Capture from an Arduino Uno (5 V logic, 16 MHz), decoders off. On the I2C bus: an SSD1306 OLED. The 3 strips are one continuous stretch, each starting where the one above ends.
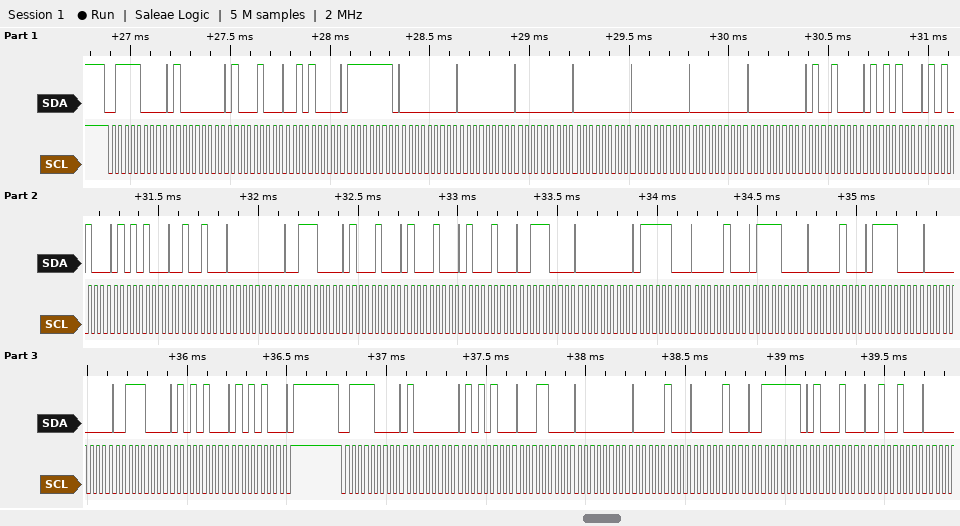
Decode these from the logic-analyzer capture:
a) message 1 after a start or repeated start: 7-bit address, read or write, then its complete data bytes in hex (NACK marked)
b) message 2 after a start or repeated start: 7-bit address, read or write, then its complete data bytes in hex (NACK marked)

0x3C write: 40 44 28 7F 00 00 00 00 00 00 00 48 54 54 54 24 00 38 44 44 44 38 00 7C 04 78 04 78 00 38 54 54
0x3C write: 40 54 18 00 04 04 3F 44 24
